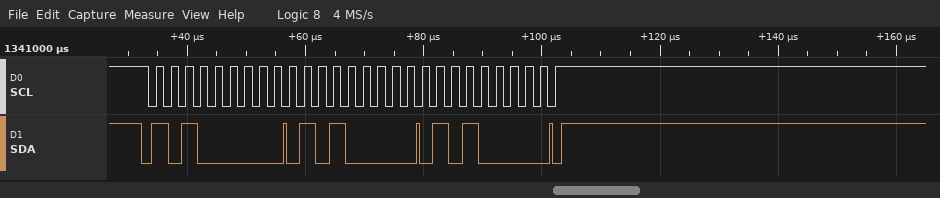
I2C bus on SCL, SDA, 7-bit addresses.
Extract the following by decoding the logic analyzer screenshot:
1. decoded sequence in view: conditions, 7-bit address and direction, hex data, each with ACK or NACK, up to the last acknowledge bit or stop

start, address 50 write ACK, 50 ACK, 50 ACK, stop
